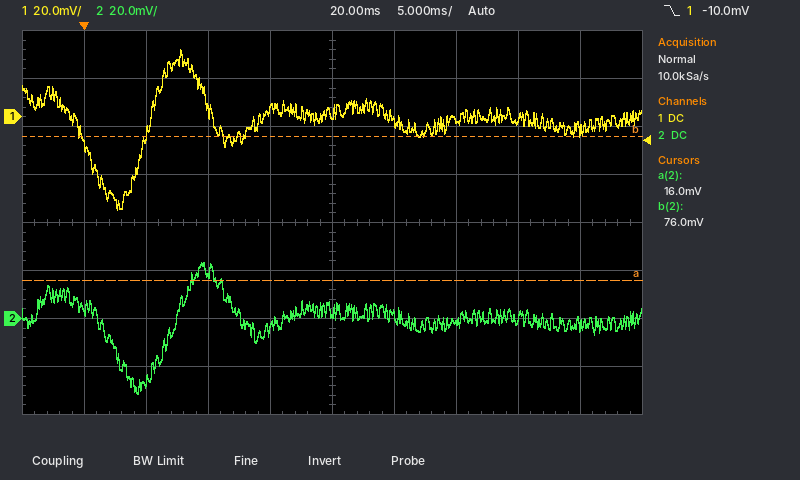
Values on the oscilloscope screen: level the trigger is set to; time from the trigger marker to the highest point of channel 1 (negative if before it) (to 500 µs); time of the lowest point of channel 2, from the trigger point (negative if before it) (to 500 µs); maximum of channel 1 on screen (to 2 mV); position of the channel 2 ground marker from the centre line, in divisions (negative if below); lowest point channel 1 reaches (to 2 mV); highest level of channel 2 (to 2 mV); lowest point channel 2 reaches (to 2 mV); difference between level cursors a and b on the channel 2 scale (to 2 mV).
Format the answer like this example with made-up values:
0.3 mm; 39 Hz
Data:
-10.0 mV; +8.0 ms; +4.5 ms; 28 mV; -2.0 div; -38 mV; 24 mV; -32 mV; 60 mV
